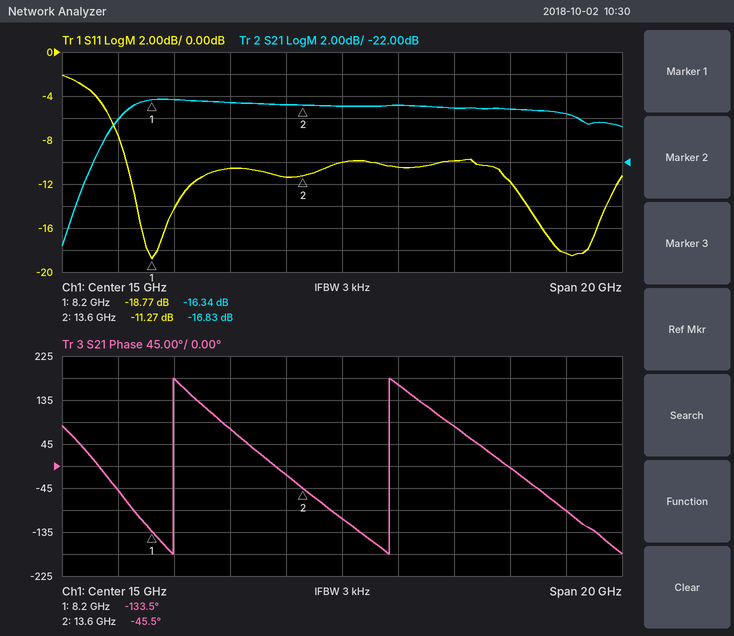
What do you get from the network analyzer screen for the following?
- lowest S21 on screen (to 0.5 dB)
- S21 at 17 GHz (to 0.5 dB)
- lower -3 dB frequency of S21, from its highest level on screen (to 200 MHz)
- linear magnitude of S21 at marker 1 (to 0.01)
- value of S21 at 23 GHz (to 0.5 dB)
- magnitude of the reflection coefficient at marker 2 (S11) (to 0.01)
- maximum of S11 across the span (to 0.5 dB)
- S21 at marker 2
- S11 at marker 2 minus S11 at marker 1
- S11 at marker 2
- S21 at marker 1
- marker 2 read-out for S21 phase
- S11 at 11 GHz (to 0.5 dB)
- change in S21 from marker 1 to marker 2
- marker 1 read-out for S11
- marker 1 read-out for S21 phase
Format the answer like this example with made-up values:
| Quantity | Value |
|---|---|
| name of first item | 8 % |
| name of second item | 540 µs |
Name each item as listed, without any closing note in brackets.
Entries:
| Quantity | Value |
|---|---|
| lowest S21 on screen | -29.5 dB |
| S21 at 17 GHz | -17.0 dB |
| lower -3 dB frequency of S21, from its highest level on screen | 6.6 GHz |
| linear magnitude of S21 at marker 1 | 0.15 |
| value of S21 at 23 GHz | -17.5 dB |
| magnitude of the reflection coefficient at marker 2 (S11) | 0.27 |
| maximum of S11 across the span | -2.0 dB |
| S21 at marker 2 | -16.83 dB |
| S11 at marker 2 minus S11 at marker 1 | 7.50 dB |
| S11 at marker 2 | -11.27 dB |
| S21 at marker 1 | -16.34 dB |
| marker 2 read-out for S21 phase | -45.5° |
| S11 at 11 GHz | -10.5 dB |
| change in S21 from marker 1 to marker 2 | -0.49 dB |
| marker 1 read-out for S11 | -18.77 dB |
| marker 1 read-out for S21 phase | -133.5° |
